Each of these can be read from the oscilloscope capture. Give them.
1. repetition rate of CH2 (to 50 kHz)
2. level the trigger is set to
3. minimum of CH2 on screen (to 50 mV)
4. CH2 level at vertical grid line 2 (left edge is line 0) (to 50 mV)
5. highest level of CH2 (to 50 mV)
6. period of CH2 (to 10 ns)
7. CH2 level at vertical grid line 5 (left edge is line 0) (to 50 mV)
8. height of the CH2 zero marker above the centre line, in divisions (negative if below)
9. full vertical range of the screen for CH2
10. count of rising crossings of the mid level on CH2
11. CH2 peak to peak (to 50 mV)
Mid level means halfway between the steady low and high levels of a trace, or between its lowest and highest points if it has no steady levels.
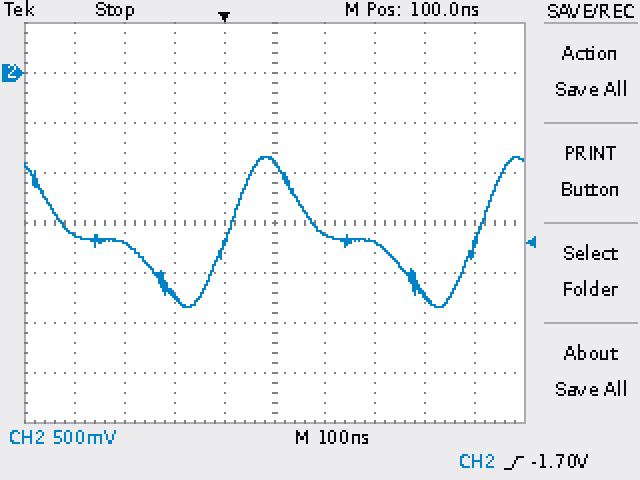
2.00 MHz
-1.70 V
-2.35 V
-1.70 V
-850 mV
500 ns
-900 mV
+3.0 div
4 V
2
1.50 V
